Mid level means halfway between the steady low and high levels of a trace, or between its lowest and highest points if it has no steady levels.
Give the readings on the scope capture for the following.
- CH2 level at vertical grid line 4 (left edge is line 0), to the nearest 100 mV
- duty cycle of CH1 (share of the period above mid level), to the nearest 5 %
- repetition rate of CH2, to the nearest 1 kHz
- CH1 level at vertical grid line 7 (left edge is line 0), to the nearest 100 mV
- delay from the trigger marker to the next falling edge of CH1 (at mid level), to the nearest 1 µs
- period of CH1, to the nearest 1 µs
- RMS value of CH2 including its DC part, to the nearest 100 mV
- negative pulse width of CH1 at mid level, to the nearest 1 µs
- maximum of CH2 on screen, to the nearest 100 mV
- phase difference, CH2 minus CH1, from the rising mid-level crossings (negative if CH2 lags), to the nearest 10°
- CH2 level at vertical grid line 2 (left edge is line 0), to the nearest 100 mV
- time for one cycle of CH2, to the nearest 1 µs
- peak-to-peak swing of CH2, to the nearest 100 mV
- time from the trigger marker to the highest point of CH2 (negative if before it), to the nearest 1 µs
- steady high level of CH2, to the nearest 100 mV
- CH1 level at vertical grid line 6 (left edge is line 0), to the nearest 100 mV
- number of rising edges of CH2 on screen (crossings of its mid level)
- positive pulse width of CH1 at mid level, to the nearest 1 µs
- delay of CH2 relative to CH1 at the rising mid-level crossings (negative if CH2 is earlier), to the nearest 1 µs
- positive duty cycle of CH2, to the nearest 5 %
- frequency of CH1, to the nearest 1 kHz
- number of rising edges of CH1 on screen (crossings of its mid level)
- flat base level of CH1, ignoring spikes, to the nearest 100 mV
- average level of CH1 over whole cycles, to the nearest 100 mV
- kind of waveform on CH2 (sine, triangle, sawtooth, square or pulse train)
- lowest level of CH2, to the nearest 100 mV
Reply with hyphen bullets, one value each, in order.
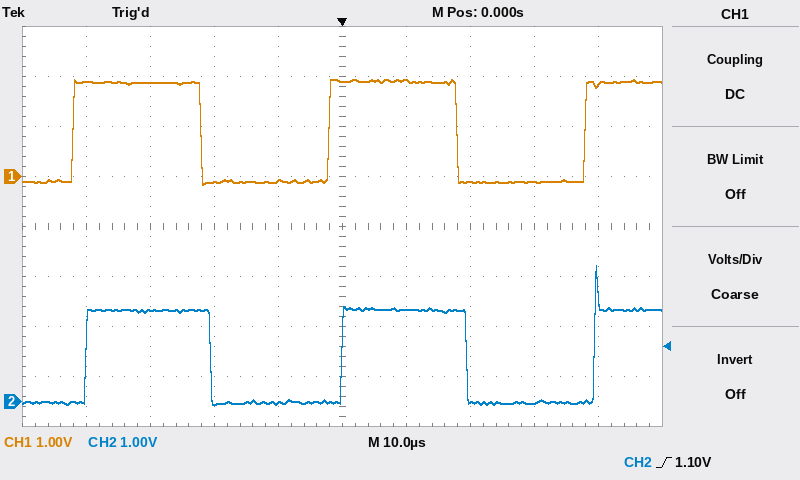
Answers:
- 0.0 V
- 50 %
- 25 kHz
- -100 mV
- 18 µs
- 40 µs
- 1.3 V
- 20 µs
- 2.7 V
- -20°
- 1.8 V
- 40 µs
- 2.8 V
- +40 µs
- 1.8 V
- 1.9 V
- 3
- 20 µs
- +2 µs
- 50 %
- 25 kHz
- 3
- -100 mV
- 900 mV
- square
- -100 mV
